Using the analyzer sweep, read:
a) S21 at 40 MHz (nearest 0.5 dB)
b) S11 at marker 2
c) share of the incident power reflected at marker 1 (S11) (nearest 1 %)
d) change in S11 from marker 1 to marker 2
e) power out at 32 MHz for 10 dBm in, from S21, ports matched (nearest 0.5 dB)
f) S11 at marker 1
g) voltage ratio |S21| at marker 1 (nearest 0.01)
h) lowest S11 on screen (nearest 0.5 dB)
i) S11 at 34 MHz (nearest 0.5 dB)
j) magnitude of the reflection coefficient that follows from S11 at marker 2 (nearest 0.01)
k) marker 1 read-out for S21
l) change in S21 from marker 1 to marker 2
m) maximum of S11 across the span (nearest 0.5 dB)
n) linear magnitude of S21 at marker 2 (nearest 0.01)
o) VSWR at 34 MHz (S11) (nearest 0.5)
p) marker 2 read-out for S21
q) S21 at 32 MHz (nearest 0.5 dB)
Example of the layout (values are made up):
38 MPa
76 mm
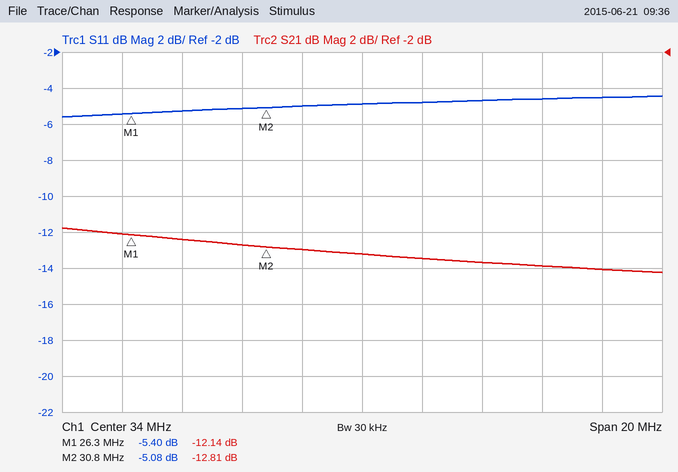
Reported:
-14.0 dB
-5.08 dB
29 %
0.32 dB
-3.0 dBm
-5.40 dB
0.25
-5.5 dB
-5.0 dB
0.56
-12.14 dB
-0.67 dB
-4.5 dB
0.23
3.5
-12.81 dB
-13.0 dB
